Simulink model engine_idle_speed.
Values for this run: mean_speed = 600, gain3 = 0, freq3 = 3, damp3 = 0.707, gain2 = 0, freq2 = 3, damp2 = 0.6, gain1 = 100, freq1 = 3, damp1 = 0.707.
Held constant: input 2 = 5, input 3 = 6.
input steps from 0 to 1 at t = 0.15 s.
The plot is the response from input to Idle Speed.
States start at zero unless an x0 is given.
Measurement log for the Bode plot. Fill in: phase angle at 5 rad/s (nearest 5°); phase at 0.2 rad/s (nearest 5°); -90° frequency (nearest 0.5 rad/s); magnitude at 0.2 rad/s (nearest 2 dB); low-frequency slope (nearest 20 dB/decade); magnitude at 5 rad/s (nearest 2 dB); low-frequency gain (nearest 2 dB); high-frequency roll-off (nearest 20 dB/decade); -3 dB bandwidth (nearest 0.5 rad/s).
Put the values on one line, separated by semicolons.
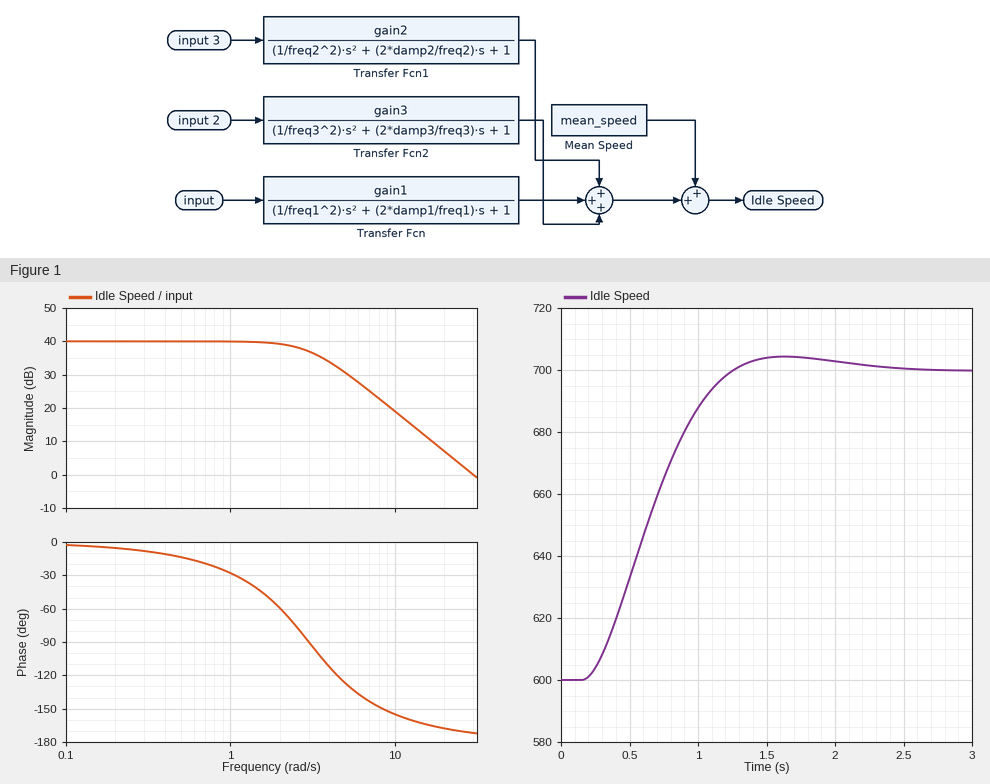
-125°; -5°; 3.0 rad/s; 40 dB; 0 dB/decade; 30 dB; 40 dB; -40 dB/decade; 3.0 rad/s
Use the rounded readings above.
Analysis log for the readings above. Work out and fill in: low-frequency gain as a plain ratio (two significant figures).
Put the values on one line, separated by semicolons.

100
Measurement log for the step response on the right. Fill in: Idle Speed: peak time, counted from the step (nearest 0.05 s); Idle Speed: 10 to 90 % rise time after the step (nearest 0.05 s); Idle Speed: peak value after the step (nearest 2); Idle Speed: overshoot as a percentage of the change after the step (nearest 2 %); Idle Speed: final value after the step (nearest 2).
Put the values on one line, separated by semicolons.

1.50 s; 0.70 s; 704; 4 %; 700
